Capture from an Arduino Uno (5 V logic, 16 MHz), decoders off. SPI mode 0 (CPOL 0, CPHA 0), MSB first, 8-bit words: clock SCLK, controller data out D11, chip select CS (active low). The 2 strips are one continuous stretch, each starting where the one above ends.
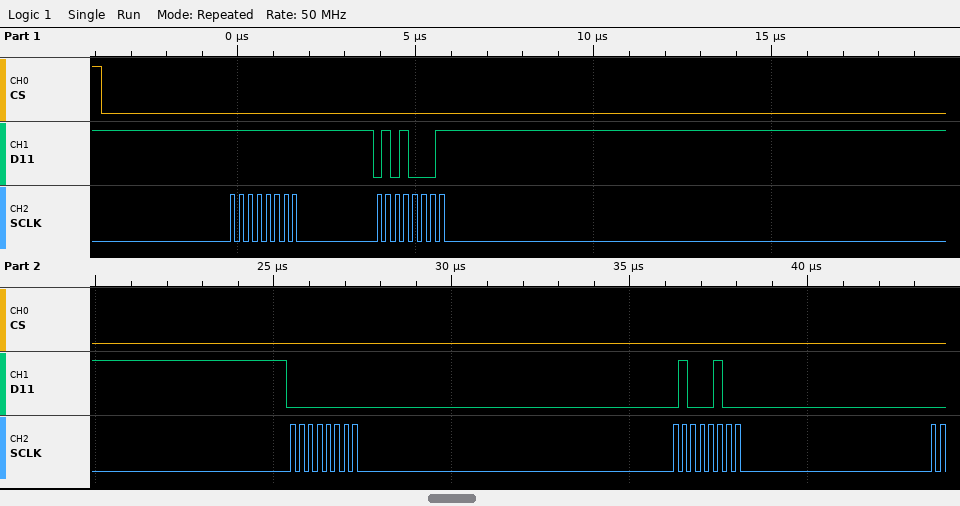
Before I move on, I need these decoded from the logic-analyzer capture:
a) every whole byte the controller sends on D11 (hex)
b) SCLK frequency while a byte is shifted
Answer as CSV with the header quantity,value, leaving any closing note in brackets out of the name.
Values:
quantity,value
every whole byte the controller sends on D11,0xFF 0x51 0x00 0x44
SCLK frequency while a byte is shifted,4 MHz
